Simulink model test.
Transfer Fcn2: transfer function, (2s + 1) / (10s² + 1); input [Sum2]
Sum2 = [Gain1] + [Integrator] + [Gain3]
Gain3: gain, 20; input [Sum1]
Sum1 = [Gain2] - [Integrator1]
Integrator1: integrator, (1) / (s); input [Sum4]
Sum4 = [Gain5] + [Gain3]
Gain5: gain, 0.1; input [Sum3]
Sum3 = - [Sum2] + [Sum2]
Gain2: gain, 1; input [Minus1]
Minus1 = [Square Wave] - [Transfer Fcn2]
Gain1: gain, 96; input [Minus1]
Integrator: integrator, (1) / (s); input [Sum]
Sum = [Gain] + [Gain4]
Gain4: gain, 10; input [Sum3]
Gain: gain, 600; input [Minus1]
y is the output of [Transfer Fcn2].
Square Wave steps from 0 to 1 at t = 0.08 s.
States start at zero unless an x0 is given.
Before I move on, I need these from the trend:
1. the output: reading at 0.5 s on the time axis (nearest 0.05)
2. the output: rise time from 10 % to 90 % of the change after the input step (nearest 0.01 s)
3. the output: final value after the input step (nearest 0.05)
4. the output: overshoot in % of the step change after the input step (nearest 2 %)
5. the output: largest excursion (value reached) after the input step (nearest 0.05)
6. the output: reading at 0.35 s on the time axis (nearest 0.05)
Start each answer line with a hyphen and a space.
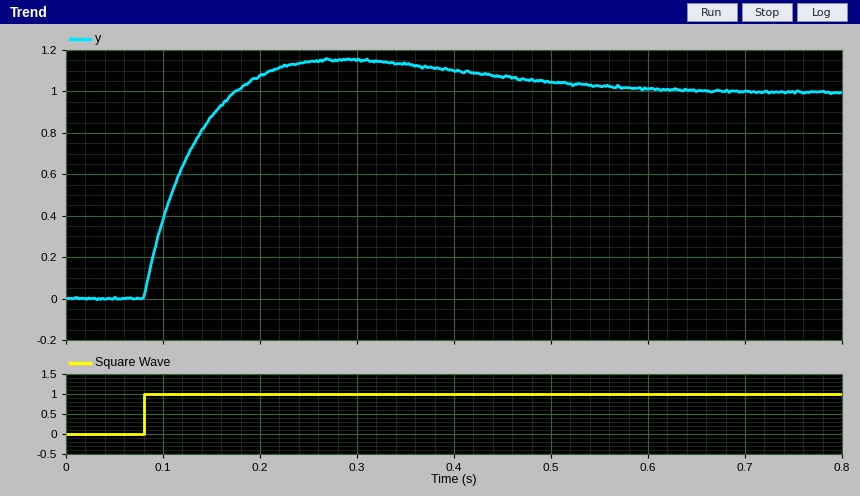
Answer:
- 1.05
- 0.07 s
- 1.00
- 16 %
- 1.15
- 1.15
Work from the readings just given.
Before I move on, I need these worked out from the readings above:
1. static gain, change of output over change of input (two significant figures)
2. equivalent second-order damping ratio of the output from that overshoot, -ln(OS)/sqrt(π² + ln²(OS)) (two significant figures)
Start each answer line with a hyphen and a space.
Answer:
- 1.0
- 0.50
